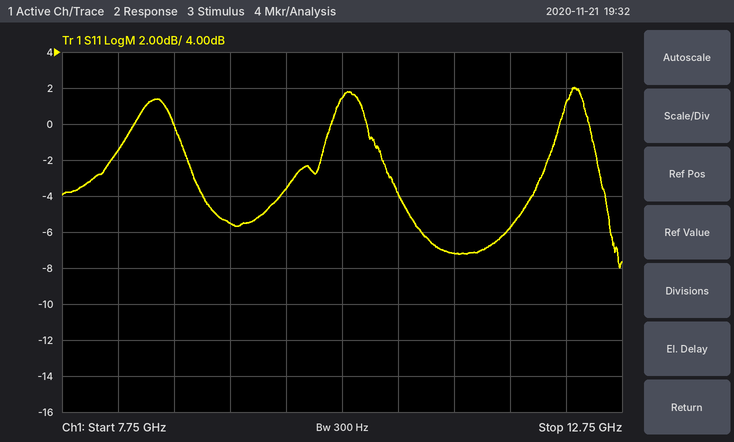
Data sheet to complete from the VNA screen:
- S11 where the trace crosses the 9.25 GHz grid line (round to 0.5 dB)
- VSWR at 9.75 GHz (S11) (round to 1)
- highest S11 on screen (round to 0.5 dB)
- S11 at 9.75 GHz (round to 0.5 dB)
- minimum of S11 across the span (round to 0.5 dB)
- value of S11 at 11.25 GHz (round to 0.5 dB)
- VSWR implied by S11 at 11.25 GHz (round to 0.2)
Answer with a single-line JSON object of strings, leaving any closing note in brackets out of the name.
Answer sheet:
{"S11 where the trace crosses the 9.25 GHz grid line": "-5.5 dB", "VSWR at 9.75 GHz (S11)": "5", "highest S11 on screen": "2.0 dB", "S11 at 9.75 GHz": "-3.5 dB", "minimum of S11 across the span": "-8.0 dB", "value of S11 at 11.25 GHz": "-7.0 dB", "VSWR implied by S11 at 11.25 GHz": "2.6"}
